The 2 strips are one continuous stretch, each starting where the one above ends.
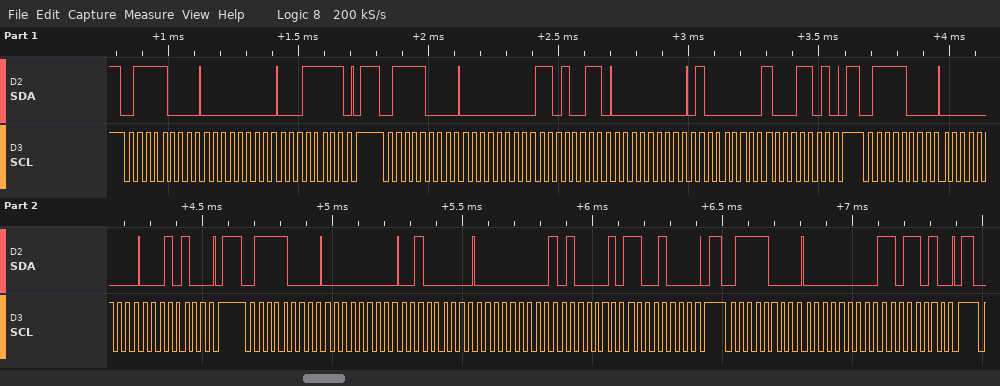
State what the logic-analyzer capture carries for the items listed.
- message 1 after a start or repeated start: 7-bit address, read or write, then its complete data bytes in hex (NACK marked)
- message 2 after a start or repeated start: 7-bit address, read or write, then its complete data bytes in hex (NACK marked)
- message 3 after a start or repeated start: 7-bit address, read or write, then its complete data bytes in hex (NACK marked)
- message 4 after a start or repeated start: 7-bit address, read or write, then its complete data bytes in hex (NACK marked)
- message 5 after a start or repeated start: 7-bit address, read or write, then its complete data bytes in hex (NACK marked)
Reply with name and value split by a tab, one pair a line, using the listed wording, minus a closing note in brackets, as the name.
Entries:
message 1 after a start or repeated start: 7-bit address, read or write, then its complete data bytes in hex	0x3C write: 00 1F
message 2 after a start or repeated start: 7-bit address, read or write, then its complete data bytes in hex	0x3C write: 00 D3 00 40 8D
message 3 after a start or repeated start: 7-bit address, read or write, then its complete data bytes in hex	0x3C write: 00 14
message 4 after a start or repeated start: 7-bit address, read or write, then its complete data bytes in hex	0x3C write: 00 20 00 A1 C8
message 5 after a start or repeated start: 7-bit address, read or write, then its complete data bytes in hex	0x3C write: 00 DA
